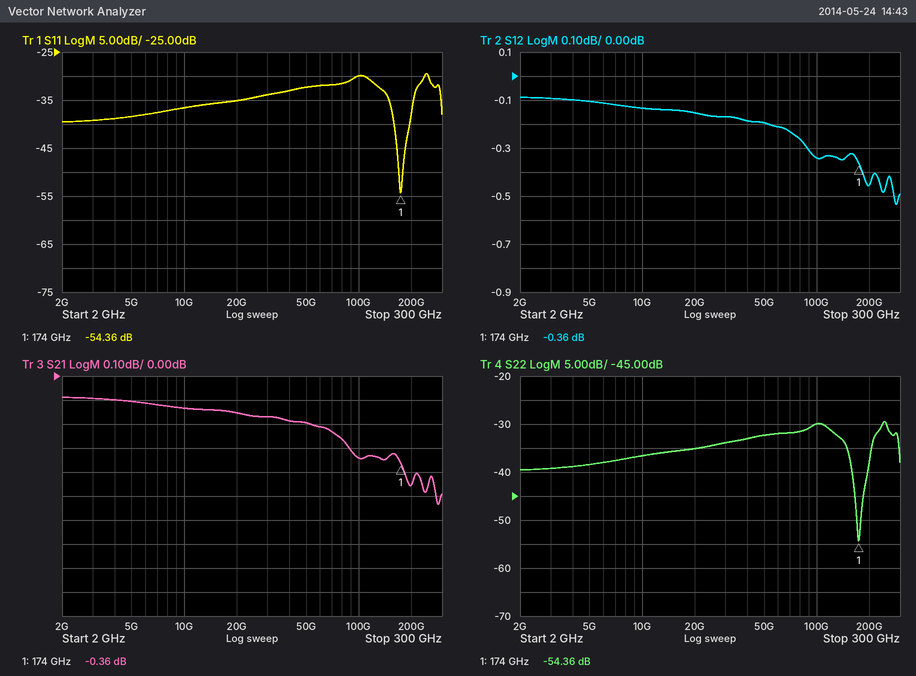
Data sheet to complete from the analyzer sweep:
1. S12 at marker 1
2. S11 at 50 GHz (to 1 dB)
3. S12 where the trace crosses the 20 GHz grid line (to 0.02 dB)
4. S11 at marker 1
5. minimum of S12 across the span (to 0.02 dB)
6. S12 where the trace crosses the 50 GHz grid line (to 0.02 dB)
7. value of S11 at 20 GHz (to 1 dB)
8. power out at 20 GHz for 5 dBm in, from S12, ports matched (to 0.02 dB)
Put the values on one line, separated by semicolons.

-0.36 dB; -32 dB; -0.16 dB; -54.36 dB; -0.54 dB; -0.20 dB; -35 dB; 4.84 dBm
